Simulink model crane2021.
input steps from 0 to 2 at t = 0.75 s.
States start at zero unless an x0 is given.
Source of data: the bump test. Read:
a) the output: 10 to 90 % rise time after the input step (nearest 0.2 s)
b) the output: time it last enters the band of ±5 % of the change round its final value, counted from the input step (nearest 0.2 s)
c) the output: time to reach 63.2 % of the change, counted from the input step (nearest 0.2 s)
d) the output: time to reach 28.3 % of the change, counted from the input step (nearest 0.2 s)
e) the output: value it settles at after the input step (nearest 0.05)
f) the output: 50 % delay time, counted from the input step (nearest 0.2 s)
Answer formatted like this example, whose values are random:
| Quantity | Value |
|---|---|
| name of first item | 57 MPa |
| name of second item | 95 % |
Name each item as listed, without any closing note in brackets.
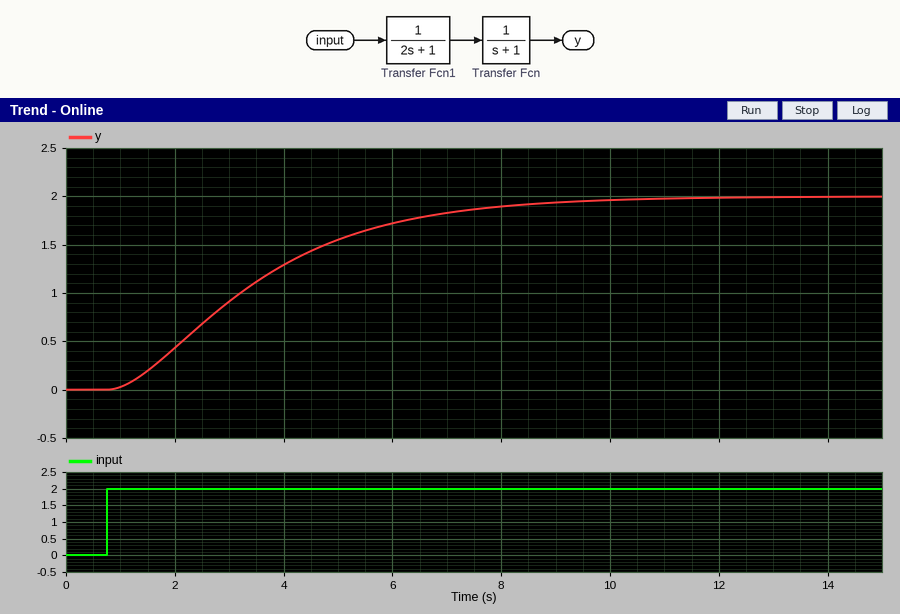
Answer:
| Quantity | Value |
|---|---|
| the output: 10 to 90 % rise time after the input step | 5.2 s |
| the output: time it last enters the band of ±5 % of the change round its final value, counted from the input step | 7.4 s |
| the output: time to reach 63.2 % of the change, counted from the input step | 3.2 s |
| the output: time to reach 28.3 % of the change, counted from the input step | 1.6 s |
| the output: value it settles at after the input step | 2.00 |
| the output: 50 % delay time, counted from the input step | 2.4 s |
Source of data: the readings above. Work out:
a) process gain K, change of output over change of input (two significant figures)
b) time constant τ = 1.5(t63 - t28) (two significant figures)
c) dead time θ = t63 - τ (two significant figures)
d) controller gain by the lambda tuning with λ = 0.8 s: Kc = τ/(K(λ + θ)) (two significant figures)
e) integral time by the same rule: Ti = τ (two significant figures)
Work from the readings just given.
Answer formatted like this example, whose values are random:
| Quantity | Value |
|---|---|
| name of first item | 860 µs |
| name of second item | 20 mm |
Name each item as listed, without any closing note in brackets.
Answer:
| Quantity | Value |
|---|---|
| process gain K, change of output over change of input | 1.0 |
| time constant τ = 1.5(t63 - t28) | 2.4 s |
| dead time θ = t63 - τ | 0.80 s |
| controller gain by the lambda tuning with λ = 0.8 s: Kc = τ/(K(λ + θ)) | 1.5 |
| integral time by the same rule: Ti = τ | 2.4 s |
